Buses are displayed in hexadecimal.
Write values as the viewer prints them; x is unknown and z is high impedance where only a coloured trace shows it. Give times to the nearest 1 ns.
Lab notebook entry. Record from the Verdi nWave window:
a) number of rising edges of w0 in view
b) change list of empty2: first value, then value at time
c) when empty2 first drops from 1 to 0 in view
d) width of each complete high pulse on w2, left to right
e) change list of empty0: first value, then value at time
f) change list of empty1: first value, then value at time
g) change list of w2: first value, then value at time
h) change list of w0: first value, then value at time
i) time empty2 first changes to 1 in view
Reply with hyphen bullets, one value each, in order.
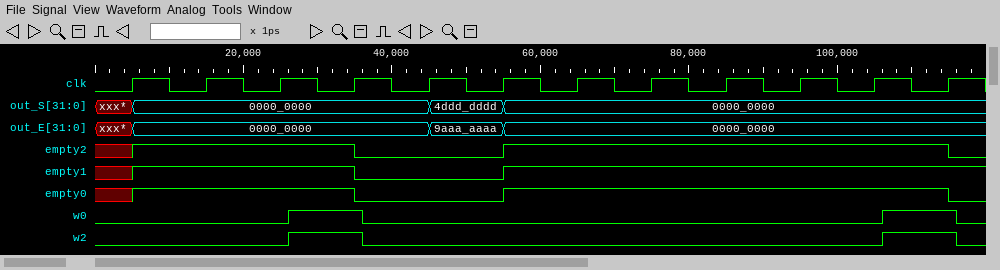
- 2
- x, 1 at 5 ns, 0 at 35 ns, 1 at 55 ns, 0 at 115 ns
- 35 ns
- 10 ns, 10 ns
- x, 1 at 5 ns, 0 at 35 ns, 1 at 55 ns, 0 at 115 ns
- x, 1 at 5 ns, 0 at 35 ns, 1 at 55 ns
- 0, 1 at 26 ns, 0 at 36 ns, 1 at 106 ns, 0 at 116 ns
- 0, 1 at 26 ns, 0 at 36 ns, 1 at 106 ns, 0 at 116 ns
- 5 ns
